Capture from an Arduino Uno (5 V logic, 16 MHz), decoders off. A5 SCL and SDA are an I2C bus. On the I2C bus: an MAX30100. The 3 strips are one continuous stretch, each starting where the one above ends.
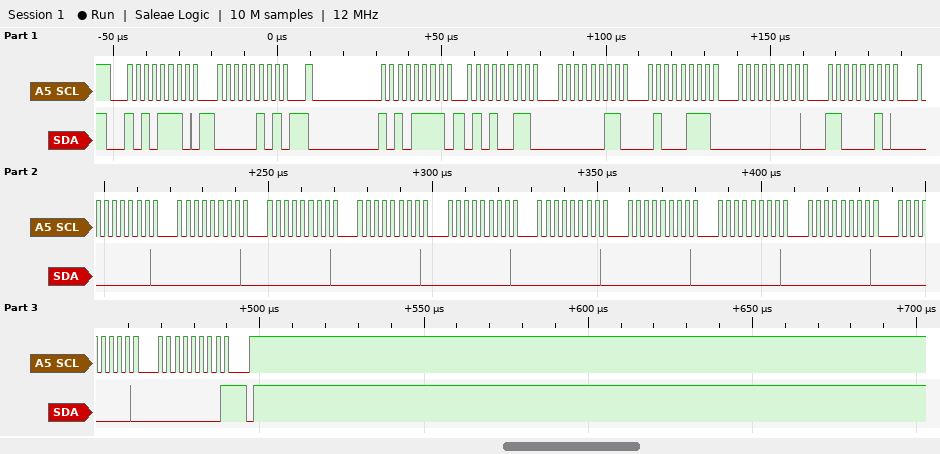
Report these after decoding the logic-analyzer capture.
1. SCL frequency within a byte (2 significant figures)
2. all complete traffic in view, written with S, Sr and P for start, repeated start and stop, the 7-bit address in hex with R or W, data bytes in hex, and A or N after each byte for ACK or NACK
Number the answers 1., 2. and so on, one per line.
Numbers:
1. 400 kHz
2. S 57W A 05 A Sr 57R A 53 A 03 A 47 A 00 A C2 A 00 A 00 A 00 A 00 A 00 A 00 A 00 A 00 A 00 A 00 A 00 N P
